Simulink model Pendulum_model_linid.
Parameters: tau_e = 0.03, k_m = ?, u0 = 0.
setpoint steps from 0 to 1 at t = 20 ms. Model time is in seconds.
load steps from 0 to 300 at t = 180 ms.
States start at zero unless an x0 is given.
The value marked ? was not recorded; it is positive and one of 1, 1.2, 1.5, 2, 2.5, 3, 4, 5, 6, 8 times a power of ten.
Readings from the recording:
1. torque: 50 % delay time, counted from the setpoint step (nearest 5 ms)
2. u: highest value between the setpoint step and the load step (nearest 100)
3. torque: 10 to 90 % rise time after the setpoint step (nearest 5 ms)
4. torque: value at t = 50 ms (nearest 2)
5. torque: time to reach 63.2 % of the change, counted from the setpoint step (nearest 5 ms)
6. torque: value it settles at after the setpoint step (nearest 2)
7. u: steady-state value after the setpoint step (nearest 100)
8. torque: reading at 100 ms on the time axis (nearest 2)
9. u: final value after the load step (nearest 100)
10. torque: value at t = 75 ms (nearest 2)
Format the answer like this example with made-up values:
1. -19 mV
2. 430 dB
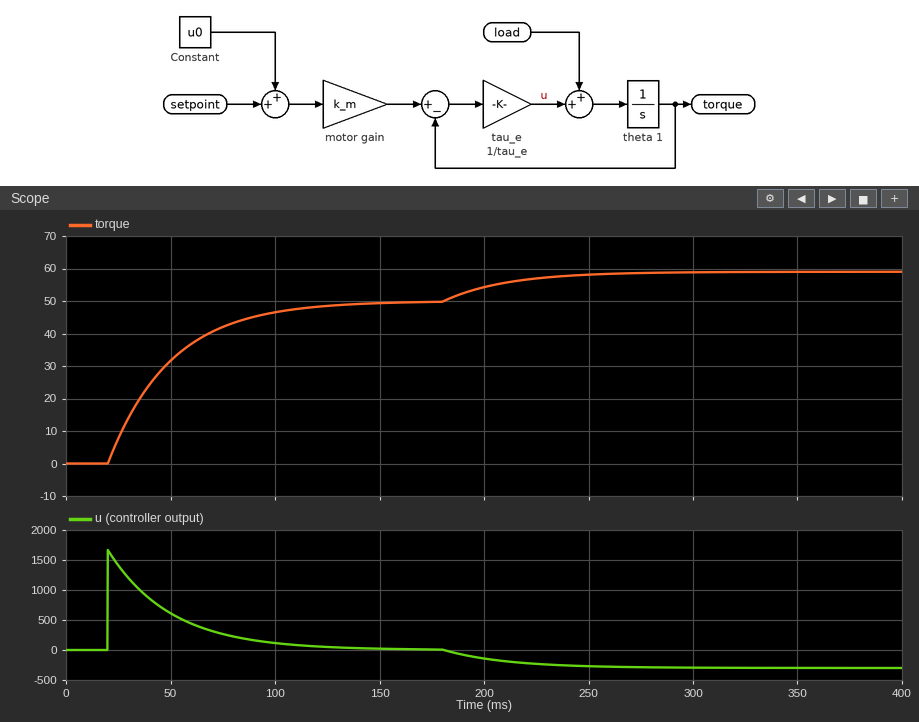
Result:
1. 20 ms
2. 1700
3. 65 ms
4. 32
5. 30 ms
6. 50
7. 0
8. 46
9. -300
10. 42
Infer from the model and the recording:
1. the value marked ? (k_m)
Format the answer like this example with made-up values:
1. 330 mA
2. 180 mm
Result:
1. 50
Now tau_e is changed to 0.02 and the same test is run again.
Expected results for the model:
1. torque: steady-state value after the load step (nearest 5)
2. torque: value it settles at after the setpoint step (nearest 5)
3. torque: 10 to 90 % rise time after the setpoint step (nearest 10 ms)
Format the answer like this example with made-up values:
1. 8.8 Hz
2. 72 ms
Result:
1. 55
2. 50
3. 40 ms
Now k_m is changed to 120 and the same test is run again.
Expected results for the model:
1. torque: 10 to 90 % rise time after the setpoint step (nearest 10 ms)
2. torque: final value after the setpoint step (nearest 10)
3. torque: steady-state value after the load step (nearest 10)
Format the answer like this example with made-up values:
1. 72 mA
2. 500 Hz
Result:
1. 70 ms
2. 120
3. 130
